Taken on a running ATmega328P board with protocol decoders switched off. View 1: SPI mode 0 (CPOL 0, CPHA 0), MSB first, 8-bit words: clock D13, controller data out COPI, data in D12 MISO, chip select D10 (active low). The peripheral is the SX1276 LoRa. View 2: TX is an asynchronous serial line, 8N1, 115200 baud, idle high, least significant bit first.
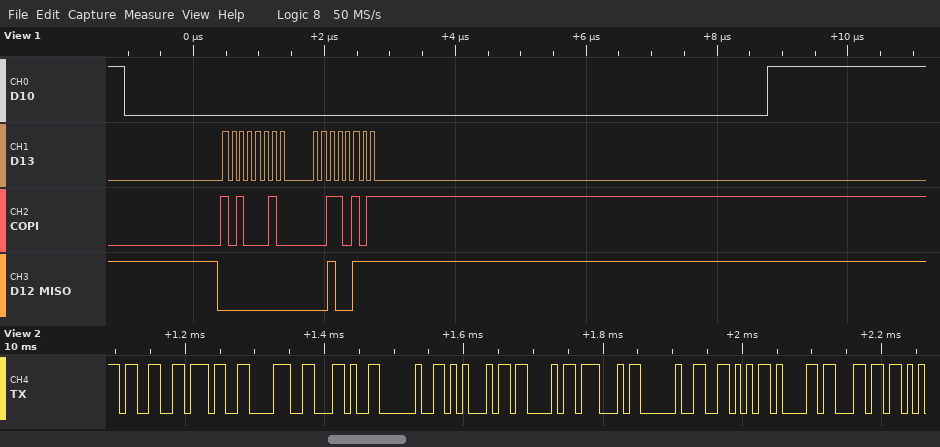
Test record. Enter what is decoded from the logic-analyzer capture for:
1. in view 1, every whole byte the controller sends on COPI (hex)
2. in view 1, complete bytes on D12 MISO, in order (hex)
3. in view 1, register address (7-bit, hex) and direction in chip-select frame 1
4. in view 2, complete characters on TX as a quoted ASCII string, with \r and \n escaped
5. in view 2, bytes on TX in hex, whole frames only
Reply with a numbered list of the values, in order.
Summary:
1. 0xA2 0x35
2. 0x00 0x27
3. 0x22 write
4. "378, ECG Val"
5. 33 37 38 2C 20 45 43 47 20 56 61 6C
